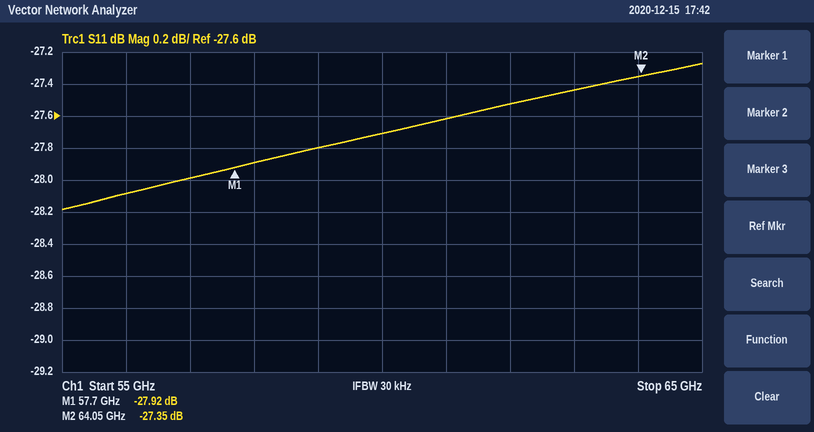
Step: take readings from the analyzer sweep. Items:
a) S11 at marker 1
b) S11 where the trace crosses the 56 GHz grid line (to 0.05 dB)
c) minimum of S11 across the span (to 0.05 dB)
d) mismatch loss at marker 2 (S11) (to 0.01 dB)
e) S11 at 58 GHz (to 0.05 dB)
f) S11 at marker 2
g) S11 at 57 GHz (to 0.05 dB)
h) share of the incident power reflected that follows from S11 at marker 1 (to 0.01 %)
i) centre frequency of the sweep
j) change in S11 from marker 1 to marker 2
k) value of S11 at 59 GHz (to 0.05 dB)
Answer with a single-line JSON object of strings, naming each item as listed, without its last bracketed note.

{"S11 at marker 1": "-27.92 dB", "S11 where the trace crosses the 56 GHz grid line": "-28.10 dB", "minimum of S11 across the span": "-28.20 dB", "mismatch loss at marker 2 (S11)": "0.01 dB", "S11 at 58 GHz": "-27.90 dB", "S11 at marker 2": "-27.35 dB", "S11 at 57 GHz": "-28.00 dB", "share of the incident power reflected that follows from S11 at marker 1": "0.16 %", "centre frequency of the sweep": "60 GHz", "change in S11 from marker 1 to marker 2": "0.57 dB", "value of S11 at 59 GHz": "-27.80 dB"}
